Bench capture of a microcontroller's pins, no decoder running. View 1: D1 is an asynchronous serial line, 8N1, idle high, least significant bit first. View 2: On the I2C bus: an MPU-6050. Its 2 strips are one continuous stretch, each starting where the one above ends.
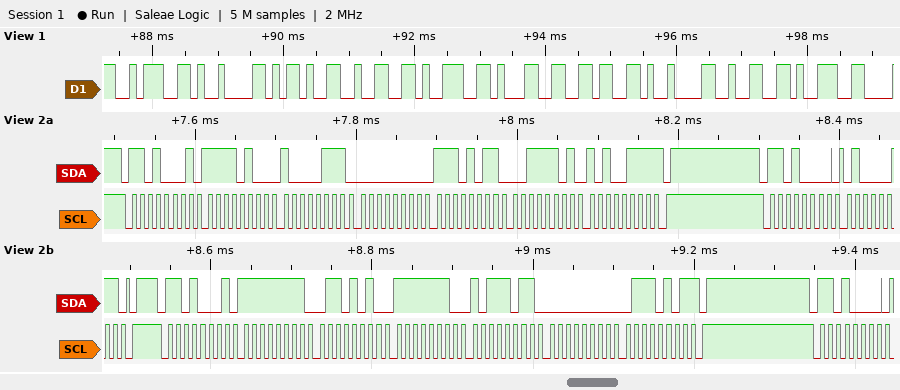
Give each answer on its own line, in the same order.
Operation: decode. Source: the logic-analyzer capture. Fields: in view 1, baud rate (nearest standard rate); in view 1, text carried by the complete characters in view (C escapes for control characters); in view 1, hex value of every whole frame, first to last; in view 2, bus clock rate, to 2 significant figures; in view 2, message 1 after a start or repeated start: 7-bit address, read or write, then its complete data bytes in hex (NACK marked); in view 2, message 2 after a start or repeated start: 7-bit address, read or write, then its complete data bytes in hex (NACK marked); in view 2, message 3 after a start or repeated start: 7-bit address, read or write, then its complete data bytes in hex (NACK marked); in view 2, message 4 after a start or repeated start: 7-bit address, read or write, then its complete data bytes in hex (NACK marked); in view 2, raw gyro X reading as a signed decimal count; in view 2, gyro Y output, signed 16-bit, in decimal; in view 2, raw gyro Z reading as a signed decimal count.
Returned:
9600 baud
":\t-2916\t29"
3A 09 2D 32 39 31 36 09 32 39
100 kHz
0x68 read: F4 87 00 EB 3D A7 NACK
0x68 write: 43
0x68 read: FF 6A FE BB 00 75 NACK
0x68 write
-150
-325
117
